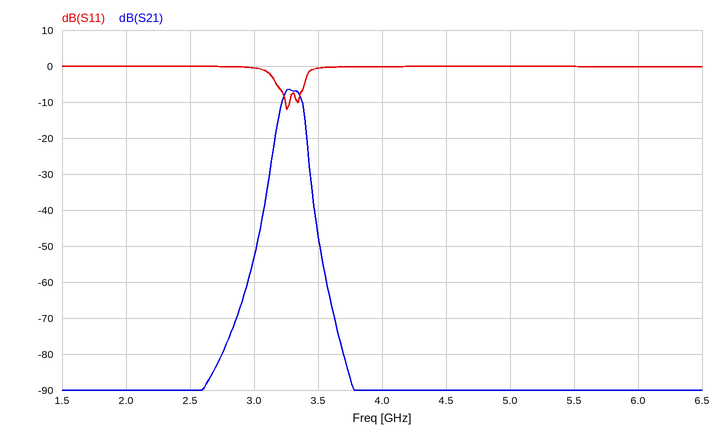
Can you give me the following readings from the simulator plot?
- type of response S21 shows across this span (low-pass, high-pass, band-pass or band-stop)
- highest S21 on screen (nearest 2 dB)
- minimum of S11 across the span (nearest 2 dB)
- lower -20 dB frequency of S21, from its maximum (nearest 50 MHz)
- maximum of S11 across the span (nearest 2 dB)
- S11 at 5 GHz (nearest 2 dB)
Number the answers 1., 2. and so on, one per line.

1. band-pass
2. -6 dB
3. -12 dB
4. 3.15 GHz
5. 0 dB
6. 0 dB
